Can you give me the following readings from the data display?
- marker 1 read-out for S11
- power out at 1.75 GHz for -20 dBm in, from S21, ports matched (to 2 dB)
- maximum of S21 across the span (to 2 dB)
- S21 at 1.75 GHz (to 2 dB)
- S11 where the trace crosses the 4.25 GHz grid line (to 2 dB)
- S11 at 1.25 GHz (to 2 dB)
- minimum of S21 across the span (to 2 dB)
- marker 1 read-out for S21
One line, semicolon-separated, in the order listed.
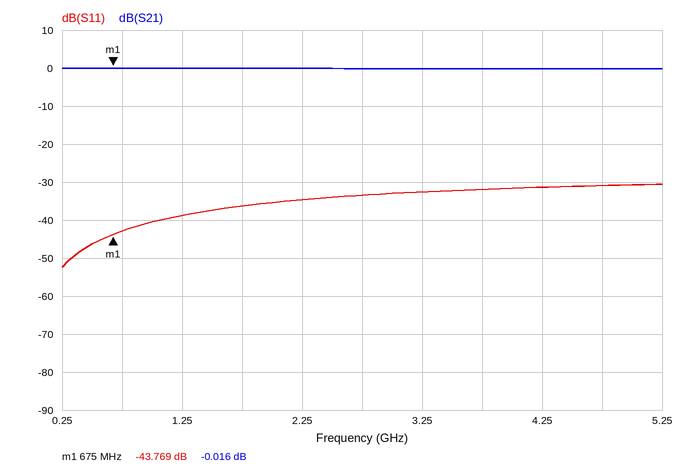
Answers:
-43.769 dB; -20 dBm; 0 dB; 0 dB; -32 dB; -38 dB; 0 dB; -0.016 dB
